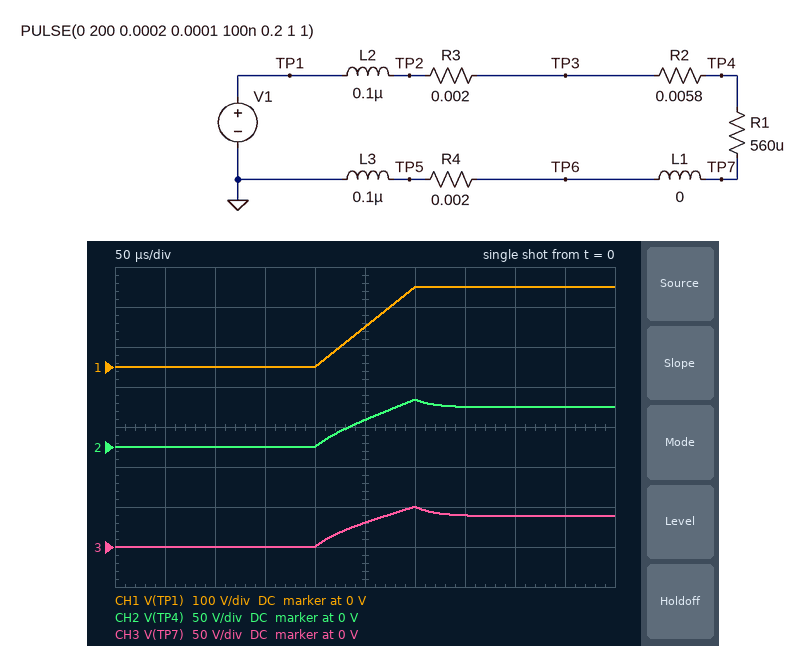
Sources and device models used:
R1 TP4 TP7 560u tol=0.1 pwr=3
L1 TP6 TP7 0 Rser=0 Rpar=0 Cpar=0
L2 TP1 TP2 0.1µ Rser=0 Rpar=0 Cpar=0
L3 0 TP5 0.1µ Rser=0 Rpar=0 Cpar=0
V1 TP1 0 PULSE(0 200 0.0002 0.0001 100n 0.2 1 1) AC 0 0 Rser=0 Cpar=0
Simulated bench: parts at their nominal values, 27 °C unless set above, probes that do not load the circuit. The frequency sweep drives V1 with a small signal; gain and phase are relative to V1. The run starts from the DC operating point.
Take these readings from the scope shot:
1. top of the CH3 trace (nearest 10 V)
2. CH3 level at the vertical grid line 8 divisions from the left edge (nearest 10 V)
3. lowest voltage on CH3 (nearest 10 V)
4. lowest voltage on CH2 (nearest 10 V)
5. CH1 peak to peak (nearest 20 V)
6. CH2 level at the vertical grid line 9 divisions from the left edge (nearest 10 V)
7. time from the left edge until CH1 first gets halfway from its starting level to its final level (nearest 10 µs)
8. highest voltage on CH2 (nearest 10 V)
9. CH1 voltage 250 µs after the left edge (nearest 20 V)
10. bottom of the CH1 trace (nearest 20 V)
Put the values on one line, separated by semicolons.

50 V; 40 V; 0 V; 0 V; 200 V; 50 V; 250 µs; 60 V; 100 V; 0 V
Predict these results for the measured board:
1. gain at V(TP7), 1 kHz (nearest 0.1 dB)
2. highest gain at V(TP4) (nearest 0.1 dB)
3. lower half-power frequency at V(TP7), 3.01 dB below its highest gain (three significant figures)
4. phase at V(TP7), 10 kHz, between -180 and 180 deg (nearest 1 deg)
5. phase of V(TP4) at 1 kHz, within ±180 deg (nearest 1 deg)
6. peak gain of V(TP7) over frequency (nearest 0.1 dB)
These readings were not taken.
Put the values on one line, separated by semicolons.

-13.9 dB; -6.0 dB; 6.91 kHz; 22 deg; 7 deg; -6.0 dB
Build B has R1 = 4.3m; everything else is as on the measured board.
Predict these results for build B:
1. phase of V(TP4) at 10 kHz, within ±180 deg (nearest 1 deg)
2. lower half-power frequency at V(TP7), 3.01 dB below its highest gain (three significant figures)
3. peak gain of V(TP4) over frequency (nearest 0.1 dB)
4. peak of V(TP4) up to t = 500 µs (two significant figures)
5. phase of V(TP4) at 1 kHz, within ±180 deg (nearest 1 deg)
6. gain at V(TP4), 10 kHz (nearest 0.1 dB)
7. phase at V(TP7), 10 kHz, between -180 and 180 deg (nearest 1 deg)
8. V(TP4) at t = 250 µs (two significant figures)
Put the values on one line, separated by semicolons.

3 deg; 10.3 kHz; -6.0 dB; 91 V; 1 deg; -6.5 dB; 31 deg; 46 V
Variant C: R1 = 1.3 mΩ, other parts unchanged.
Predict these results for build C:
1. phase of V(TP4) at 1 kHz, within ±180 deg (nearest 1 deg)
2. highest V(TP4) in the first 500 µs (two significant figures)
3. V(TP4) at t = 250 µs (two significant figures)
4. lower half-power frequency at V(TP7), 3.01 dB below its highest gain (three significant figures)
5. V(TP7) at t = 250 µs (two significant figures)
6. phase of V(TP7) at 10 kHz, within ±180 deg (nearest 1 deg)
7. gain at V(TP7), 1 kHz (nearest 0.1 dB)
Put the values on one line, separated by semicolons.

4 deg; 67 V; 37 V; 7.60 kHz; 29 V; 24 deg; -14.5 dB
